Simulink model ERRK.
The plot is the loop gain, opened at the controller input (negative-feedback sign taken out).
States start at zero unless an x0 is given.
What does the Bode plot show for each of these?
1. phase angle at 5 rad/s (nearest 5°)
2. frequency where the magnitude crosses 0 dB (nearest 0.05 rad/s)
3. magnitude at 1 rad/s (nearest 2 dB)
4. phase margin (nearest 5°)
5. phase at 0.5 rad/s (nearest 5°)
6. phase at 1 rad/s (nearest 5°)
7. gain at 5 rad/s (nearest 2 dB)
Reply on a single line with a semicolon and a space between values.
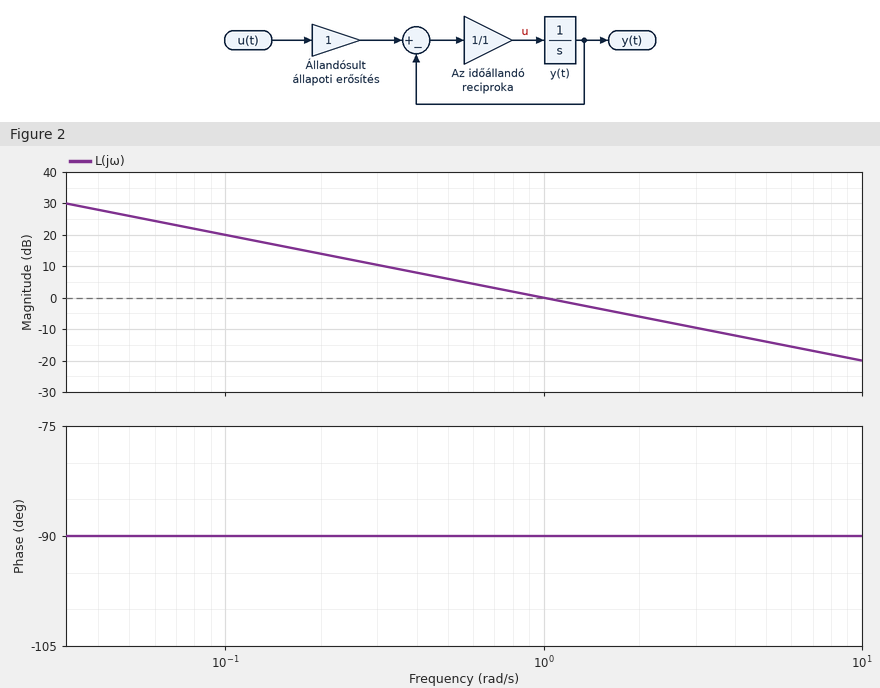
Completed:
-90°; 1.00 rad/s; 0 dB; 90°; -90°; -90°; -14 dB
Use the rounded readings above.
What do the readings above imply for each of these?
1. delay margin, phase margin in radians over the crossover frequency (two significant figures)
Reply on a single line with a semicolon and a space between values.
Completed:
1.6 s
